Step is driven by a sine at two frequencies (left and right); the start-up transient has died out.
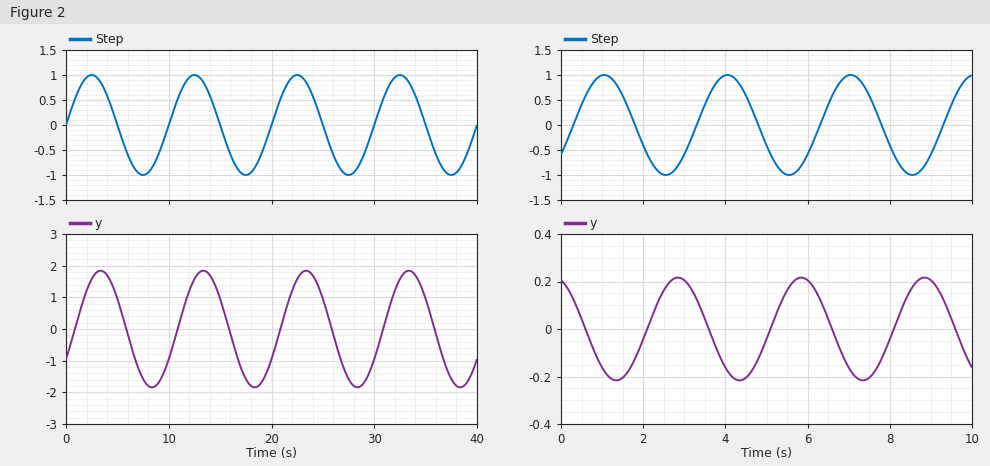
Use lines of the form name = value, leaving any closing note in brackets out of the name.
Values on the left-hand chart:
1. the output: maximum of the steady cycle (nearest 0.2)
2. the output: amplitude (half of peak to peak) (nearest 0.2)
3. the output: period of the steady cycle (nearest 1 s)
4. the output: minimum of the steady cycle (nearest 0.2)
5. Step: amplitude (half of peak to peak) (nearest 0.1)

the output: maximum of the steady cycle = 1.8
the output: amplitude (half of peak to peak) = 1.8
the output: period of the steady cycle = 10 s
the output: minimum of the steady cycle = -1.8
Step: amplitude (half of peak to peak) = 1.0
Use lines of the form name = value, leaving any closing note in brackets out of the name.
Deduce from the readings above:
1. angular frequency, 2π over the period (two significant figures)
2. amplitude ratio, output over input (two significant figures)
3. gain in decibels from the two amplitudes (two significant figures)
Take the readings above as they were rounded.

angular frequency, 2π over the period = 0.63 rad/s
amplitude ratio, output over input = 1.8
gain in decibels from the two amplitudes = 5.1 dB
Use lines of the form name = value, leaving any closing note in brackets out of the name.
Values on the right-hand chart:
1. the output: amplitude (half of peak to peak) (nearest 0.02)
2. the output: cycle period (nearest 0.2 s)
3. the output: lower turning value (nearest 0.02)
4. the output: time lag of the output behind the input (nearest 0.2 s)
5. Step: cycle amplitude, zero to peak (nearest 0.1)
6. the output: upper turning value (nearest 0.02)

the output: amplitude (half of peak to peak) = 0.22
the output: cycle period = 3.0 s
the output: lower turning value = -0.22
the output: time lag of the output behind the input = 1.8 s
Step: cycle amplitude, zero to peak = 1.0
the output: upper turning value = 0.22
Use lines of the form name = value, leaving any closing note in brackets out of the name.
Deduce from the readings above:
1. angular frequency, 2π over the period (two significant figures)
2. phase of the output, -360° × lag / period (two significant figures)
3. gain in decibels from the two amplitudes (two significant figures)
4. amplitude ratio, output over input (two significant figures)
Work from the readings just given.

angular frequency, 2π over the period = 2.1 rad/s
phase of the output, -360° × lag / period = -220°
gain in decibels from the two amplitudes = -13 dB
amplitude ratio, output over input = 0.22
